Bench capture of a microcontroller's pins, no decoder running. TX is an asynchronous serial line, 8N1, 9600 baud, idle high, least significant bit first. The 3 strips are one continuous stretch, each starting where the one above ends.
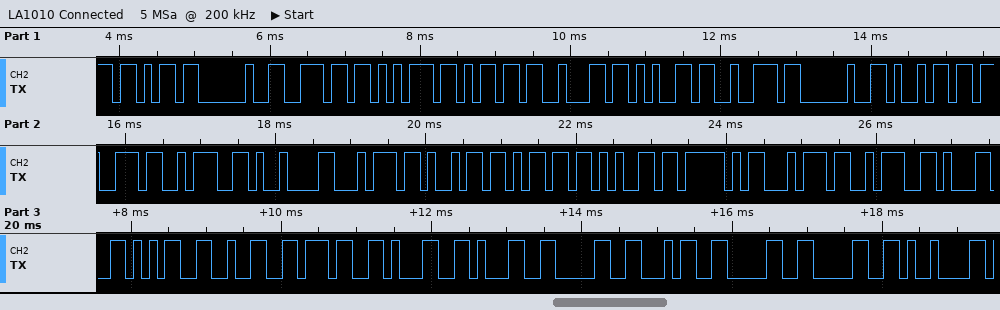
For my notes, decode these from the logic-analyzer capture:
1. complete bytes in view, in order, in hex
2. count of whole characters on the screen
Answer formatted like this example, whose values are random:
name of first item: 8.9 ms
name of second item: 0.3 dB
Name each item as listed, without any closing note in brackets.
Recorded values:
complete bytes in view, in order, in hex: 0x6B 0x20 0x6E 0x75 0x6D 0x62 0x65 0x72 0x20 0x69 0x73 0x3A 0x09 0x74 0x69 0x6D 0x65 0x5F 0x74 0x3A 0x31 0x35 0x32 0x37 0x31 0x31 0x30 0x34 0x30 0x30 0x09
count of whole characters on the screen: 31
